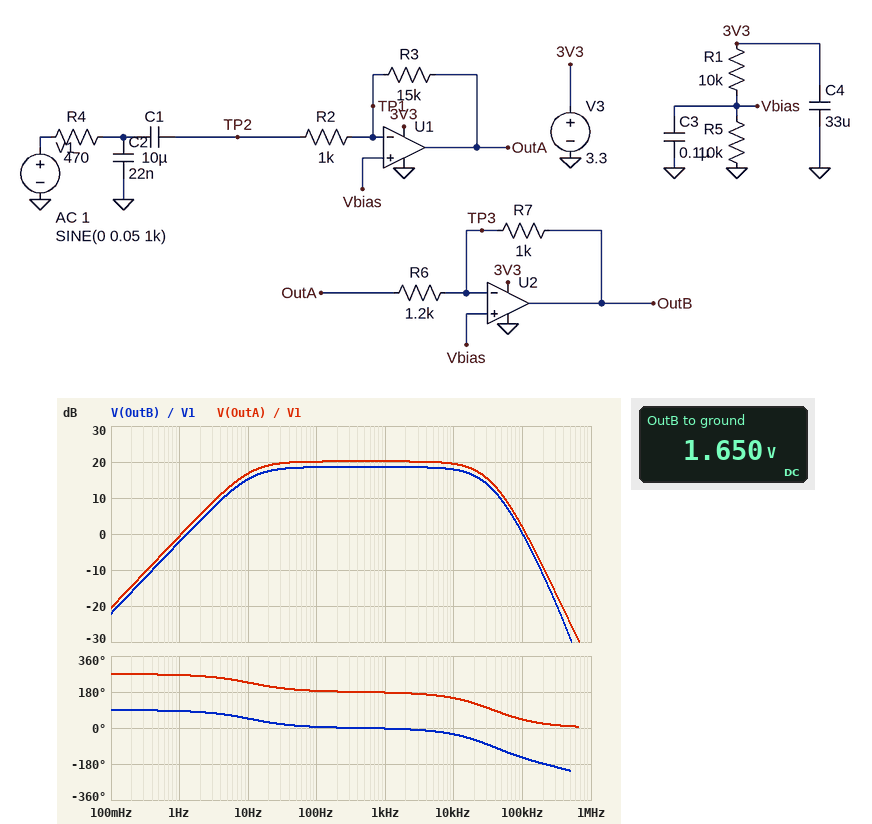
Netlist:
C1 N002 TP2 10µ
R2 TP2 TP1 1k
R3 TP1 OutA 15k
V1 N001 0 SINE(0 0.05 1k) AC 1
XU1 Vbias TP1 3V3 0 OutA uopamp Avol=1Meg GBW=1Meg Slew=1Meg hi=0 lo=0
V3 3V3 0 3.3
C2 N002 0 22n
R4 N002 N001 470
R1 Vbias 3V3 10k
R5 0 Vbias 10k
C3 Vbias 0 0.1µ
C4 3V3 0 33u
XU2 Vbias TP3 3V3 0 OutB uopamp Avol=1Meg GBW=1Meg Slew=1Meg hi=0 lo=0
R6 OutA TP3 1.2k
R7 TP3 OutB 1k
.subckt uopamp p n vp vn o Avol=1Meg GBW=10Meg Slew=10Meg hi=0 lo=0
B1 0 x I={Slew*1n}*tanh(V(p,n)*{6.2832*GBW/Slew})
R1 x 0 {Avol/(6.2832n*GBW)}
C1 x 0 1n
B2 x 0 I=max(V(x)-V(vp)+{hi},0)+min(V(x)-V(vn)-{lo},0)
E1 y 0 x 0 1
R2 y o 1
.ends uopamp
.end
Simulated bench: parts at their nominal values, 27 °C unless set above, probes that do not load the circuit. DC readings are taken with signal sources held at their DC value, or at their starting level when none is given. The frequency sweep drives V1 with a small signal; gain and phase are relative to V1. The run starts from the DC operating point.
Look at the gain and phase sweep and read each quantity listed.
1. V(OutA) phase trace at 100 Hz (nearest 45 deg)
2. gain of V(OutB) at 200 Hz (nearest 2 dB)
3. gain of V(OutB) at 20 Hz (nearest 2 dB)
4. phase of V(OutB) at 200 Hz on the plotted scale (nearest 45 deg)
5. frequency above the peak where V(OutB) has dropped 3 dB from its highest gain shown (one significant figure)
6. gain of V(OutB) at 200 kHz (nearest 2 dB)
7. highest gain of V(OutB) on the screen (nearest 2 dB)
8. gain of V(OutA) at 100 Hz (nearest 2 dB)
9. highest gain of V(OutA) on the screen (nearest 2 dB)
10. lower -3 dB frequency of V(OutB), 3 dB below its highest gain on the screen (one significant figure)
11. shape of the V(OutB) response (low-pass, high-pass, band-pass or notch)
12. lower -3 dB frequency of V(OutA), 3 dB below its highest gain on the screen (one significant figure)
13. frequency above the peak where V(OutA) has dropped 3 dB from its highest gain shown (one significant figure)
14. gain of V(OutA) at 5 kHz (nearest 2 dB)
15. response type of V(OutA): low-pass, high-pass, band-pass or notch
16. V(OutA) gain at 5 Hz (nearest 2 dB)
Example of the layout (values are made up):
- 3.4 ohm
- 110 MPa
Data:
- 180 deg
- 18 dB
- 18 dB
- 0 deg
- 20 kHz
- -12 dB
- 18 dB
- 20 dB
- 20 dB
- 10 Hz
- band-pass
- 10 Hz
- 20 kHz
- 20 dB
- band-pass
- 12 dB
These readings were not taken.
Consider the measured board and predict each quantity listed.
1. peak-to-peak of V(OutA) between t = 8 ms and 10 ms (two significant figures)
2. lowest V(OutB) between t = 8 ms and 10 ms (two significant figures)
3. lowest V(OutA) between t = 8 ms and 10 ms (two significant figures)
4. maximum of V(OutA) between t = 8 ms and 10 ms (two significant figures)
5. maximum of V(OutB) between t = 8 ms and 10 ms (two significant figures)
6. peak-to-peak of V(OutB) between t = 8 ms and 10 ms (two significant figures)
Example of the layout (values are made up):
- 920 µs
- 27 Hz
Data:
- 1.0 V
- 1.2 V
- 1.1 V
- 2.2 V
- 2.1 V
- 850 mV
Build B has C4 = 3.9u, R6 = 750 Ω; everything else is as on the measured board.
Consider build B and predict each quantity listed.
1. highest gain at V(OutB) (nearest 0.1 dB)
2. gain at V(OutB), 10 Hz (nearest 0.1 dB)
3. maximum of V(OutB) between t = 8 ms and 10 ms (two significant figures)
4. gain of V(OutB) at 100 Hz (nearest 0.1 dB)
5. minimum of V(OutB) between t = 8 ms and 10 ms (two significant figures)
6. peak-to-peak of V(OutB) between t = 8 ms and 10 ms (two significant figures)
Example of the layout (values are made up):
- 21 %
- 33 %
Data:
- 22.7 dB
- 19.3 dB
- 2.3 V
- 22.6 dB
- 970 mV
- 1.4 V
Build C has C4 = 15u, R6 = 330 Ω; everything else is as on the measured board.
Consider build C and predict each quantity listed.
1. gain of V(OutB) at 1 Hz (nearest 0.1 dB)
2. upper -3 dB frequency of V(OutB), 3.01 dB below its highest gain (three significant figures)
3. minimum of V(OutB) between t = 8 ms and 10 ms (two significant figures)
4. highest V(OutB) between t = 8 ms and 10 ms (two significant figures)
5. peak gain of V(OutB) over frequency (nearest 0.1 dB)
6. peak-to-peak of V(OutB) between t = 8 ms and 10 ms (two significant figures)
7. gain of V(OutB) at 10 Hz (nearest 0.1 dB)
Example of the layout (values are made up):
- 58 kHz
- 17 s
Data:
- 9.1 dB
- 22.7 kHz
- 96 mV
- 3.2 V
- 29.8 dB
- 3.1 V
- 26.4 dB
